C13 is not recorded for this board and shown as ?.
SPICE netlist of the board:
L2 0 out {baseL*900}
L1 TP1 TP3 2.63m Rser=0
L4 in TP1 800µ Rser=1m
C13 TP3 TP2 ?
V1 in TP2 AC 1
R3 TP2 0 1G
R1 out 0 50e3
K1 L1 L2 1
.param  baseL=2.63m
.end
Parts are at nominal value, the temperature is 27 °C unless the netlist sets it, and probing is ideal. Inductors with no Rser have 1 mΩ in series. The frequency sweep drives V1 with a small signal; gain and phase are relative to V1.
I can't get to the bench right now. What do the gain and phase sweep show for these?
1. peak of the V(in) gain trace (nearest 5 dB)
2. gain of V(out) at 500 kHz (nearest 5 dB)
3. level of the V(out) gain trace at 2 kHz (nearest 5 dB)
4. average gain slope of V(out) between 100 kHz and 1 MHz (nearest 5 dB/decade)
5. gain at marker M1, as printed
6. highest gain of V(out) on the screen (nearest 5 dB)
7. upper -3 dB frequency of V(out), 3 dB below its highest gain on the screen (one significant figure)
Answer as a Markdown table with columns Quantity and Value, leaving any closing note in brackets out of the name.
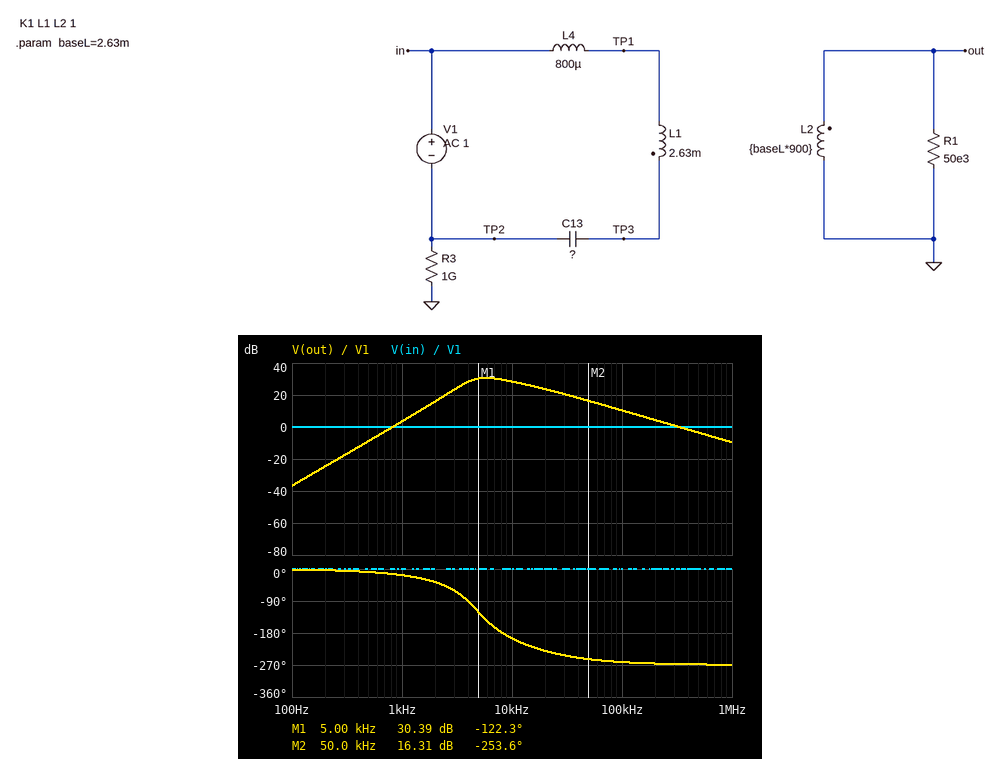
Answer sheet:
| Quantity | Value |
|---|---|
| peak of the V(in) gain trace | 0 dB |
| gain of V(out) at 500 kHz | -5 dB |
| level of the V(out) gain trace at 2 kHz | 15 dB |
| average gain slope of V(out) between 100 kHz and 1 MHz | -20 dB/decade |
| gain at marker M1, as printed | 30.39 dB |
| highest gain of V(out) on the screen | 30 dB |
| upper -3 dB frequency of V(out), 3 dB below its highest gain on the screen | 10 kHz |
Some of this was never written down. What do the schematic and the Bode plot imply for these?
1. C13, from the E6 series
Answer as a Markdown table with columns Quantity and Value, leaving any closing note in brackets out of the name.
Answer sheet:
| Quantity | Value |
|---|---|
| C13, from the E6 series | 470 nF |
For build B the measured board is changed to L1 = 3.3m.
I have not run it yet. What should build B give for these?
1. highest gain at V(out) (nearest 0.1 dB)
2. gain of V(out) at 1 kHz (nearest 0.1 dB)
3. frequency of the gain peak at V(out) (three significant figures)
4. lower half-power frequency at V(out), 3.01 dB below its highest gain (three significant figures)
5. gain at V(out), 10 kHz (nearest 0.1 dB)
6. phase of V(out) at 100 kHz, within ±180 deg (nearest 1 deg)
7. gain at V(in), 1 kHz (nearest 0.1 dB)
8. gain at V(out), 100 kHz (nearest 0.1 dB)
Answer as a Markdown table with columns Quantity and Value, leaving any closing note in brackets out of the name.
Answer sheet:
| Quantity | Value |
|---|---|
| highest gain at V(out) | 30.0 dB |
| gain of V(out) at 1 kHz | 4.6 dB |
| frequency of the gain peak at V(out) | 5.10 kHz |
| lower half-power frequency at V(out), 3.01 dB below its highest gain | 3.39 kHz |
| gain at V(out), 10 kHz | 27.7 dB |
| phase of V(out) at 100 kHz, within ±180 deg | 100 deg |
| gain at V(in), 1 kHz | 0 dB |
| gain at V(out), 100 kHz | 11.3 dB |
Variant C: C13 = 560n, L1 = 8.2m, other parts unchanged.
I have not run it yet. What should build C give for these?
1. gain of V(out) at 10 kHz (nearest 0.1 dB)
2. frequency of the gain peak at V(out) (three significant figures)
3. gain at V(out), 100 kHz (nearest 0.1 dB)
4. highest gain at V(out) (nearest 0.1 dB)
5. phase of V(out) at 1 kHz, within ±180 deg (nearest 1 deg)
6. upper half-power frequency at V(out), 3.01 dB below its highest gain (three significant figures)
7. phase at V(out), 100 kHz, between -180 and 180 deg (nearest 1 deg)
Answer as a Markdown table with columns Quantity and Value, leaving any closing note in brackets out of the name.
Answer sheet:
| Quantity | Value |
|---|---|
| gain of V(out) at 10 kHz | 24.2 dB |
| frequency of the gain peak at V(out) | 2.54 kHz |
| gain at V(out), 100 kHz | 14.8 dB |
| highest gain at V(out) | 28.7 dB |
| phase of V(out) at 1 kHz, within ±180 deg | -20 deg |
| upper half-power frequency at V(out), 3.01 dB below its highest gain | 4.76 kHz |
| phase at V(out), 100 kHz, between -180 and 180 deg | 111 deg |
